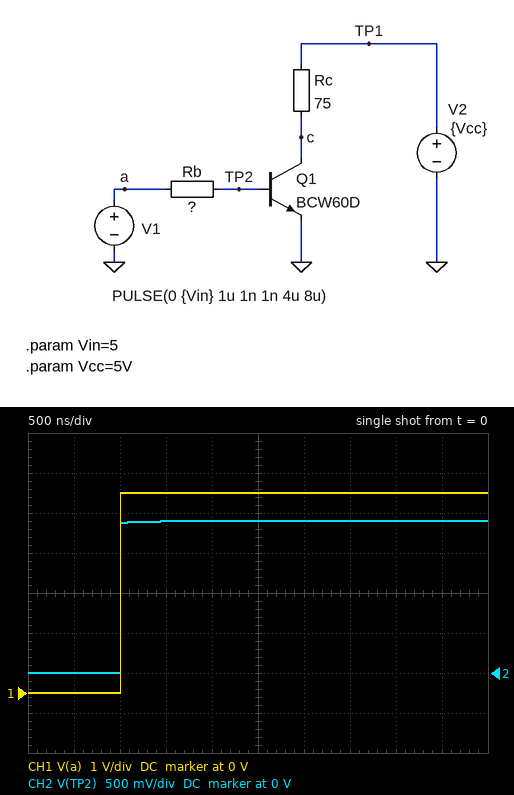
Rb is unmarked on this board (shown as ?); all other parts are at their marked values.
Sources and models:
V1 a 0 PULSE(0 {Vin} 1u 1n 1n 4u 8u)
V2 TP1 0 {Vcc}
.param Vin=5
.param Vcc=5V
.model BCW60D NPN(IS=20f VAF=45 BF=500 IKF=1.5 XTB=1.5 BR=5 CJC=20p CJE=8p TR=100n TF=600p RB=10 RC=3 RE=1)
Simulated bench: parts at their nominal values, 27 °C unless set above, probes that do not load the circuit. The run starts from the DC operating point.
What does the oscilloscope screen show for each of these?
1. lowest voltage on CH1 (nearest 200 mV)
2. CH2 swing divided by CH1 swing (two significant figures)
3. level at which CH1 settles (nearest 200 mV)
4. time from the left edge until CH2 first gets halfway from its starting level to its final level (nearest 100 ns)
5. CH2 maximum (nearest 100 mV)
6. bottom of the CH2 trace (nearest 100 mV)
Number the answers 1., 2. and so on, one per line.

1. 0 V
2. 0.38
3. 5.0 V
4. 1.0 µs
5. 1.9 V
6. 0 V
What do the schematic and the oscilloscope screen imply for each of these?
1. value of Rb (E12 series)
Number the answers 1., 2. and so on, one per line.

1. 33 Ω
